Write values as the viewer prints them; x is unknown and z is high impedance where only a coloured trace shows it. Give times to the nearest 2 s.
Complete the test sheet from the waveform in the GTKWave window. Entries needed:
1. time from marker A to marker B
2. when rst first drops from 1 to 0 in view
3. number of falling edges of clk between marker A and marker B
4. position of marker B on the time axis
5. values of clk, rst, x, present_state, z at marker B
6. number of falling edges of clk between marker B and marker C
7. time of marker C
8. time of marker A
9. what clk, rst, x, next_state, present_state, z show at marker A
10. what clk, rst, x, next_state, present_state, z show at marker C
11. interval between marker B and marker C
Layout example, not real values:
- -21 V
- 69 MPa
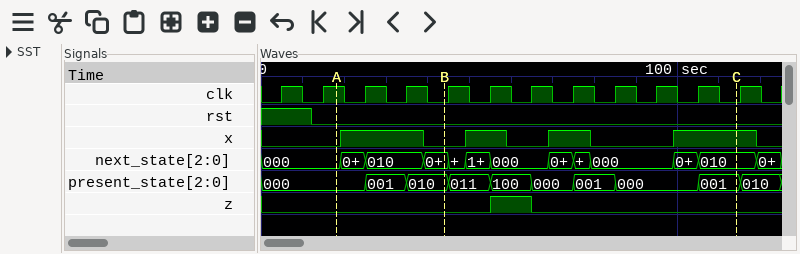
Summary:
- 26 s
- 12 s
- 3
- 44 s
- clk=0, rst=0, x=0, present_state=010, z=0
- 7
- 114 s
- 18 s
- clk=1, rst=0, x=0, next_state=000, present_state=000, z=0
- clk=0, rst=0, x=1, next_state=010, present_state=001, z=0
- 70 s
